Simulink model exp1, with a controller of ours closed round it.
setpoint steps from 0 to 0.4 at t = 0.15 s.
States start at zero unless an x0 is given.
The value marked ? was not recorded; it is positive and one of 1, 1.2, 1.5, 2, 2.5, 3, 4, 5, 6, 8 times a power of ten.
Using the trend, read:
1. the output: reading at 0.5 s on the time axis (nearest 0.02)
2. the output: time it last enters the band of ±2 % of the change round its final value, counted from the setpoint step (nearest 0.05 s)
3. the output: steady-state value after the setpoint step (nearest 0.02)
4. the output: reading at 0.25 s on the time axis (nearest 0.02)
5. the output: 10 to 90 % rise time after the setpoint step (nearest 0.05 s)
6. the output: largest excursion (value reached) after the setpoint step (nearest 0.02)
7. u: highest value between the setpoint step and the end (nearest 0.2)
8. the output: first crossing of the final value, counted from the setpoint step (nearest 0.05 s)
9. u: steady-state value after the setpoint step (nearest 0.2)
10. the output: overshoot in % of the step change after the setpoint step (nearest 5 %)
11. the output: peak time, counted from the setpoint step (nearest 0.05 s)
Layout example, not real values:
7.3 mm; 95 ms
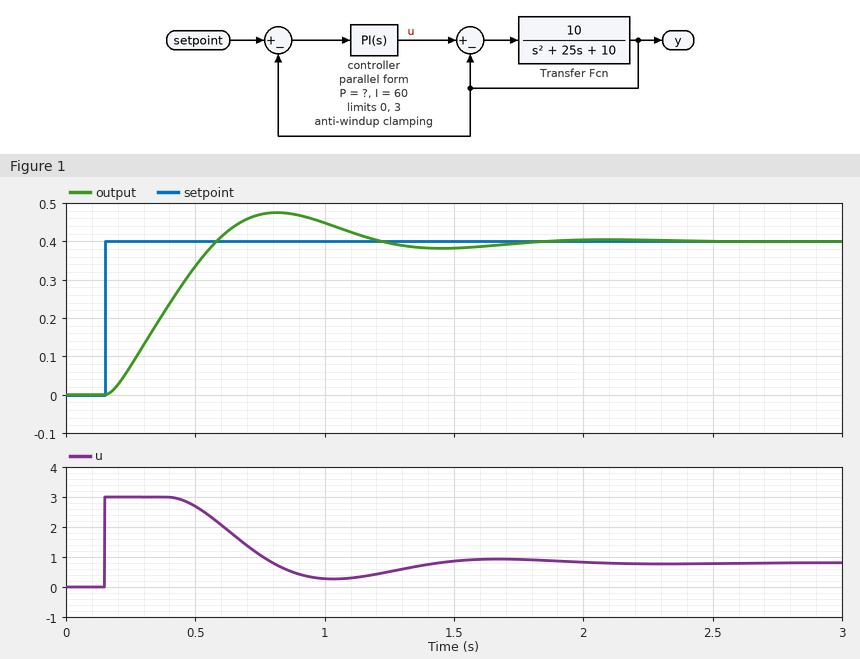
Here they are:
0.34; 1.55 s; 0.40; 0.08; 0.30 s; 0.48; 3.0; 0.45 s; 0.8; 20 %; 0.65 s
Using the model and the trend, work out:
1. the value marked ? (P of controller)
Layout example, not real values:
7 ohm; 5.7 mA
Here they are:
10
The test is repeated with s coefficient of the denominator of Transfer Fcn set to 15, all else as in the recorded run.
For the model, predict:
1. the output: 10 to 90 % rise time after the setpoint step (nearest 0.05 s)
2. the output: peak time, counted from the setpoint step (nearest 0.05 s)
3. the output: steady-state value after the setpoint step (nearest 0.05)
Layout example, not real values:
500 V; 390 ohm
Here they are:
0.20 s; 0.45 s; 0.40
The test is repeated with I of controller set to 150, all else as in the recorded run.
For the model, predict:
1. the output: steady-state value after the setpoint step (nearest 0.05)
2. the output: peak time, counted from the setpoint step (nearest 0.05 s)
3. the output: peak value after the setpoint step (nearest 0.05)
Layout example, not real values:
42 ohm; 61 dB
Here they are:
0.40; 0.60 s; 0.50
